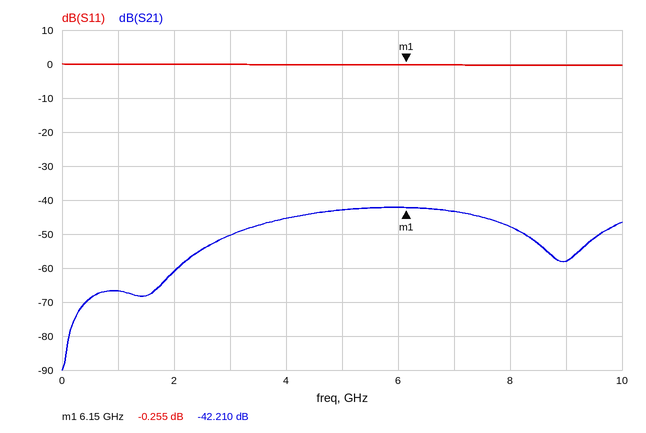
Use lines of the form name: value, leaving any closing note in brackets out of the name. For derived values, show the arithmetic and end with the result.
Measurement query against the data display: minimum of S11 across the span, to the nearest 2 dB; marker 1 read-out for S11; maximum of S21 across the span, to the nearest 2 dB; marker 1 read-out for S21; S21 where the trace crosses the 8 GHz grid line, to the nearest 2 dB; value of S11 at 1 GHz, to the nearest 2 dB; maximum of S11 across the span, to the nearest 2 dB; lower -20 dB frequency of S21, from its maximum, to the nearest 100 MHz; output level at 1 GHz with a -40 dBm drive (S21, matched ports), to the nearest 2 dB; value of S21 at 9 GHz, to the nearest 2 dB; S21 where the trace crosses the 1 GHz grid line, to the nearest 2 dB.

minimum of S11 across the span, to the nearest 2 dB: 0 dB
marker 1 read-out for S11: -0.255 dB
maximum of S21 across the span, to the nearest 2 dB: -42 dB
marker 1 read-out for S21: -42.210 dB
S21 where the trace crosses the 8 GHz grid line, to the nearest 2 dB: -48 dB
value of S11 at 1 GHz, to the nearest 2 dB: 0 dB
maximum of S11 across the span, to the nearest 2 dB: 0 dB
lower -20 dB frequency of S21, from its maximum, to the nearest 100 MHz: 1.9 GHz
output level at 1 GHz with a -40 dBm drive (S21, matched ports), to the nearest 2 dB: -40 dBm + (-66 dB) = -106 dBm
value of S21 at 9 GHz, to the nearest 2 dB: -58 dB
S21 where the trace crosses the 1 GHz grid line, to the nearest 2 dB: -66 dB
